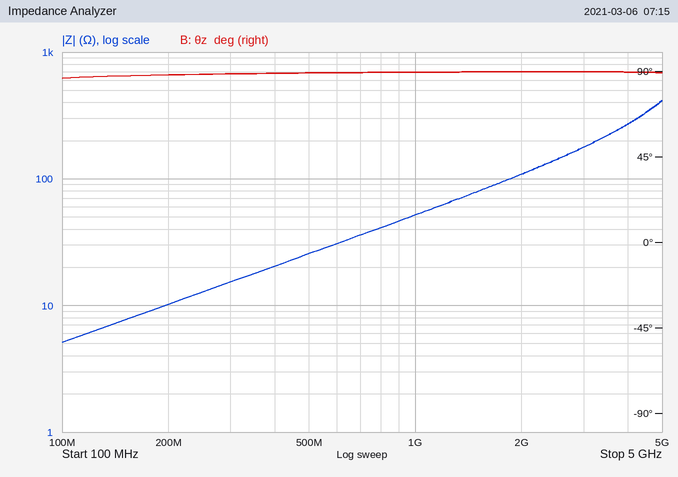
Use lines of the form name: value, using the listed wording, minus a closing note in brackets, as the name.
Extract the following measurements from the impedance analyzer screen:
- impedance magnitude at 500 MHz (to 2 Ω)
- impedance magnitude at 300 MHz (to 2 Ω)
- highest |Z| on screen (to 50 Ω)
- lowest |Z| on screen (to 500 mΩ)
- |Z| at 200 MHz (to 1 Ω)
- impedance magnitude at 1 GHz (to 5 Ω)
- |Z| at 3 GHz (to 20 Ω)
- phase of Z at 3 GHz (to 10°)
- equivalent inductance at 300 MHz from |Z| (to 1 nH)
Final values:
impedance magnitude at 500 MHz: 26 Ω
impedance magnitude at 300 MHz: 16 Ω
highest |Z| on screen: 400 Ω
lowest |Z| on screen: 5.0 Ω
|Z| at 200 MHz: 10 Ω
impedance magnitude at 1 GHz: 50 Ω
|Z| at 3 GHz: 180 Ω
phase of Z at 3 GHz: 90°
equivalent inductance at 300 MHz from |Z|: 8 nH
